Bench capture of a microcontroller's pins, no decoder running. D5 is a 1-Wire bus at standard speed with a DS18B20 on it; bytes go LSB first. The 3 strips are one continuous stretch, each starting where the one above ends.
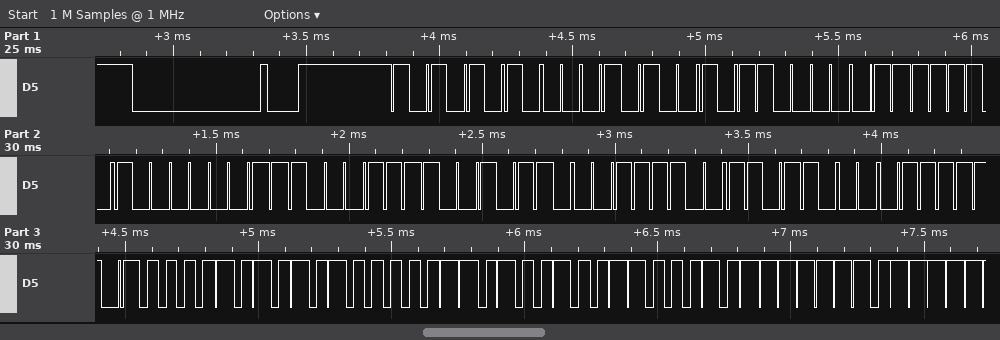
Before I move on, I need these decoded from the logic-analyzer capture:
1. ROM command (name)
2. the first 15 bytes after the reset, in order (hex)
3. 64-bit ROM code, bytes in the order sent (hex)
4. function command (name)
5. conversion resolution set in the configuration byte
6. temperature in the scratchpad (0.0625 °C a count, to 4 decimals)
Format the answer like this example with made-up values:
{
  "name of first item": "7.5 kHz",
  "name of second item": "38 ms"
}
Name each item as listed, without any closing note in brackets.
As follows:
{
  "ROM command": "Match ROM",
  "the first 15 bytes after the reset, in order": "55 28 0D 7E 81 E3 69 3C 1B BE 50 05 4B 46 7F",
  "64-bit ROM code, bytes in the order sent": "28 0D 7E 81 E3 69 3C 1B",
  "function command": "Read Scratchpad",
  "conversion resolution set in the configuration byte": "12 bits",
  "temperature in the scratchpad": "85.0000 °C"
}
